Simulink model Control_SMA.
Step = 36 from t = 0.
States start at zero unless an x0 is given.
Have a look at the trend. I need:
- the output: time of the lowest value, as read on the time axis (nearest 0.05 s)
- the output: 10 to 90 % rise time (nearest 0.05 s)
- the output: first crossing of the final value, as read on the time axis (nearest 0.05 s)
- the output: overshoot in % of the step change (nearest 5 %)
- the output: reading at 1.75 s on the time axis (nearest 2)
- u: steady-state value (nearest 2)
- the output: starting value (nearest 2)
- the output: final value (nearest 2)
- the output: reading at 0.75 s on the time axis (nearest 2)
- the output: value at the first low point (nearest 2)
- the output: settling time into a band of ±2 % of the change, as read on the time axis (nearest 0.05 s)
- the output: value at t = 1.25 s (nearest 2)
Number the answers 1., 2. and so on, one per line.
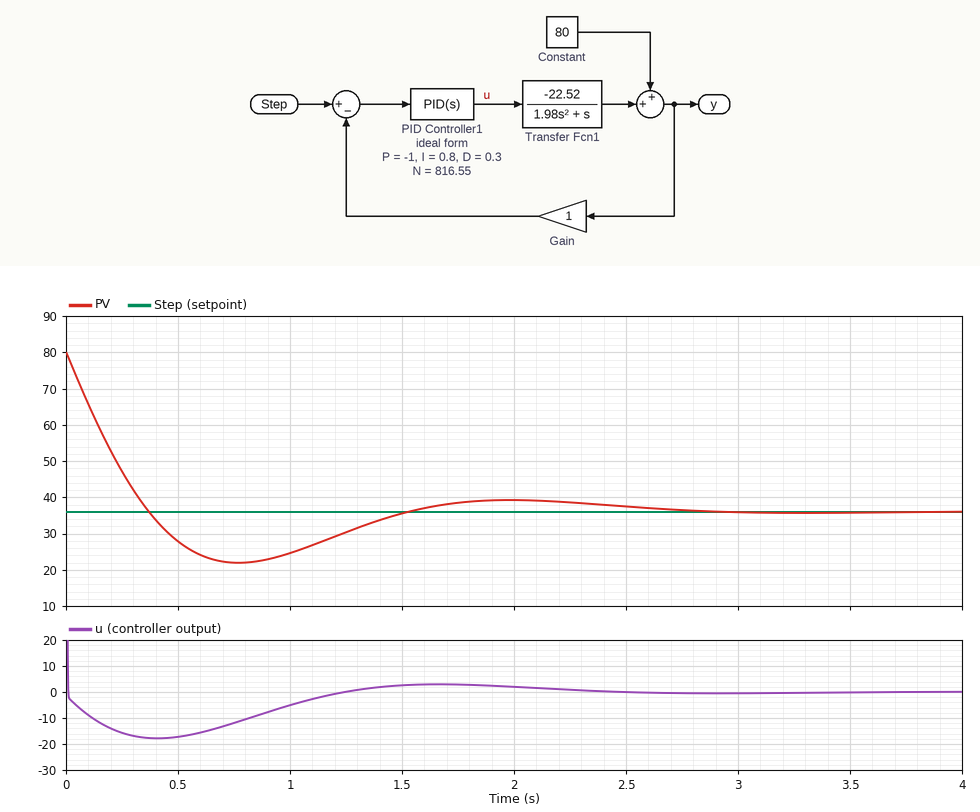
1. 0.75 s
2. 0.30 s
3. 0.35 s
4. 30 %
5. 38
6. 0
7. 80
8. 36
9. 22
10. 22
11. 2.65 s
12. 30
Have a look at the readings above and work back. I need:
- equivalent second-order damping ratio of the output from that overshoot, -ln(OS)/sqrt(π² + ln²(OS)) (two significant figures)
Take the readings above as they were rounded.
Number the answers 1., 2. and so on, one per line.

1. 0.36
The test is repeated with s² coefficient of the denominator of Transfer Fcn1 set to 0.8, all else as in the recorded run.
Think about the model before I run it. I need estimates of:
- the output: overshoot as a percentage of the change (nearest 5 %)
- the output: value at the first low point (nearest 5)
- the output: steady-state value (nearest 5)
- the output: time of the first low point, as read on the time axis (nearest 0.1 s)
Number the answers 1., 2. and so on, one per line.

1. 15 %
2. 30
3. 35
4. 0.5 s
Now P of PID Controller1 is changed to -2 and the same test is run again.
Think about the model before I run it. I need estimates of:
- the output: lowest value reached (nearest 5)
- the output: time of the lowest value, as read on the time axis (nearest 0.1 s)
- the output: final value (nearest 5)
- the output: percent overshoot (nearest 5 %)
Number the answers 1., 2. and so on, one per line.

1. 25
2. 0.5 s
3. 35
4. 20 %
